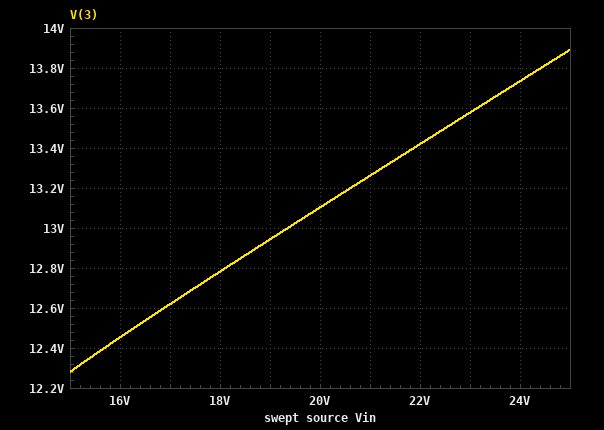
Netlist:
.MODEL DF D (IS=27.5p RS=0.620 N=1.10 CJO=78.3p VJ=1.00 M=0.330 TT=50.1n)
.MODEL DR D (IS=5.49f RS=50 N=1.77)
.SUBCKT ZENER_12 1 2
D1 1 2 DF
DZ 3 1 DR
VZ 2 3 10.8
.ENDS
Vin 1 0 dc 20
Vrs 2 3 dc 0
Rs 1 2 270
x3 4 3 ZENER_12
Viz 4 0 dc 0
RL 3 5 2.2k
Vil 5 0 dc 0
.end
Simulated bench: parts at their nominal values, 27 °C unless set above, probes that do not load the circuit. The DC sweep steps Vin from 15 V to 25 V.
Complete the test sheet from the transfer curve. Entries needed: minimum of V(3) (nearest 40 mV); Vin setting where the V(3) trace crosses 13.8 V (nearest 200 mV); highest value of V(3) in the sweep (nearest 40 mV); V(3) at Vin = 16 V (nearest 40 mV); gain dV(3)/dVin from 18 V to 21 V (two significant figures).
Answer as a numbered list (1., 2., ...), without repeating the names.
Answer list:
1. 12.28 V
2. 24.4 V
3. 13.88 V
4. 12.44 V
5. 0.16 V/V
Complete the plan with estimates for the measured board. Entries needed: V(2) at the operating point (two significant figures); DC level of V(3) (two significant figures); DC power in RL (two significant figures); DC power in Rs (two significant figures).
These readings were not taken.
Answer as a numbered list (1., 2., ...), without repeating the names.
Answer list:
1. 13 V
2. 13 V
3. 78 mW
4. 180 mW
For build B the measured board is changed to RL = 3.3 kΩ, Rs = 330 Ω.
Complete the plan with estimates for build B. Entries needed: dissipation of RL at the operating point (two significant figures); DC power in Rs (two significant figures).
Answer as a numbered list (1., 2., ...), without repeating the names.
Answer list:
1. 51 mW
2. 150 mW
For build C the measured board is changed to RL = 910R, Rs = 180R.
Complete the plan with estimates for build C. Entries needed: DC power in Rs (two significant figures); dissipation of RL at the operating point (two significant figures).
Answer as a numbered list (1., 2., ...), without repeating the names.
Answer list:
1. 250 mW
2. 190 mW
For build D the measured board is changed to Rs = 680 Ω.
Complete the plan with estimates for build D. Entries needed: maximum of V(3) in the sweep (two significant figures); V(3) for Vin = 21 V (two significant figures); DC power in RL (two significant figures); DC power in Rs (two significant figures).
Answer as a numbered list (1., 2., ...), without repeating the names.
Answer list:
1. 13 V
2. 12 V
3. 69 mW
4. 86 mW
